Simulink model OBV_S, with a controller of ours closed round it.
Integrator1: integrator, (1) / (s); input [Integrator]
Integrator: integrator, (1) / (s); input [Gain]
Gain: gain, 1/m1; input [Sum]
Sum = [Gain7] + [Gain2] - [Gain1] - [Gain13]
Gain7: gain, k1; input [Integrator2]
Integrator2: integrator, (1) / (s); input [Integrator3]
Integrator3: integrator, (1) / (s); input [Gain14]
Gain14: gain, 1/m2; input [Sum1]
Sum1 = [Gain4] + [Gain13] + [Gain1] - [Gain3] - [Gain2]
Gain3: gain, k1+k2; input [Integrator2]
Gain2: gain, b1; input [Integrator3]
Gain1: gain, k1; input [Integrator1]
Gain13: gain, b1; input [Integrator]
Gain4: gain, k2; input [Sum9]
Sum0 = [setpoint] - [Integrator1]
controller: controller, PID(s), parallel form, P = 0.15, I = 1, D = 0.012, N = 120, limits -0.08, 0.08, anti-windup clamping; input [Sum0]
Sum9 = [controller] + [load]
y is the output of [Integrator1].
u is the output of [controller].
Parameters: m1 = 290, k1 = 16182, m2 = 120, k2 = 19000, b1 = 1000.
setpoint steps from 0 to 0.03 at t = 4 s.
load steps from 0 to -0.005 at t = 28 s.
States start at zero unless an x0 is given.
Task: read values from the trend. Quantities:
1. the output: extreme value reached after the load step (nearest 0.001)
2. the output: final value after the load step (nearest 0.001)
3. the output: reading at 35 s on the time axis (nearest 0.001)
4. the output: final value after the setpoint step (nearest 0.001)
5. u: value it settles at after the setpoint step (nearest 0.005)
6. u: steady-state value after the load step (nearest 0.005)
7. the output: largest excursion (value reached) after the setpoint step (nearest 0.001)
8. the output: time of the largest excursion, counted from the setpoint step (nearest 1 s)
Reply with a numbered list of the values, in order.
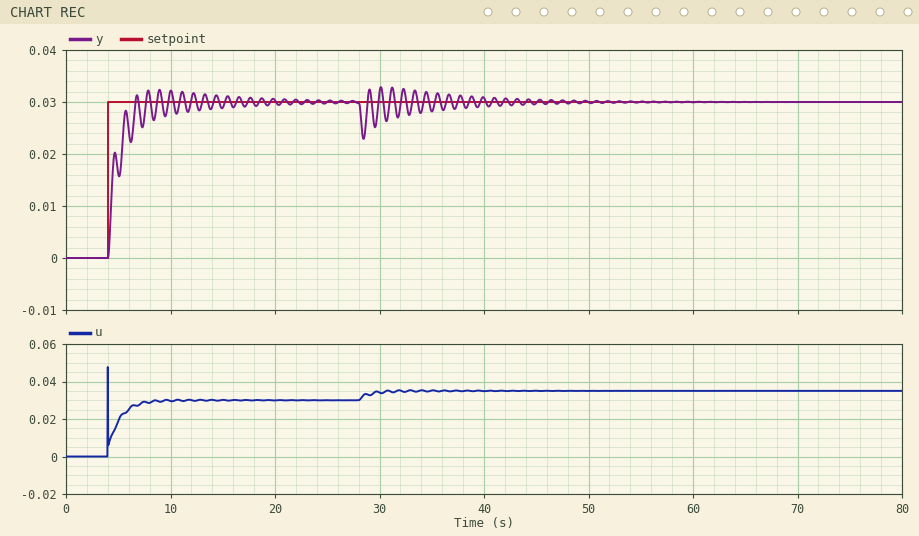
1. 0.023
2. 0.030
3. 0.028
4. 0.030
5. 0.030
6. 0.035
7. 0.032
8. 5 s
